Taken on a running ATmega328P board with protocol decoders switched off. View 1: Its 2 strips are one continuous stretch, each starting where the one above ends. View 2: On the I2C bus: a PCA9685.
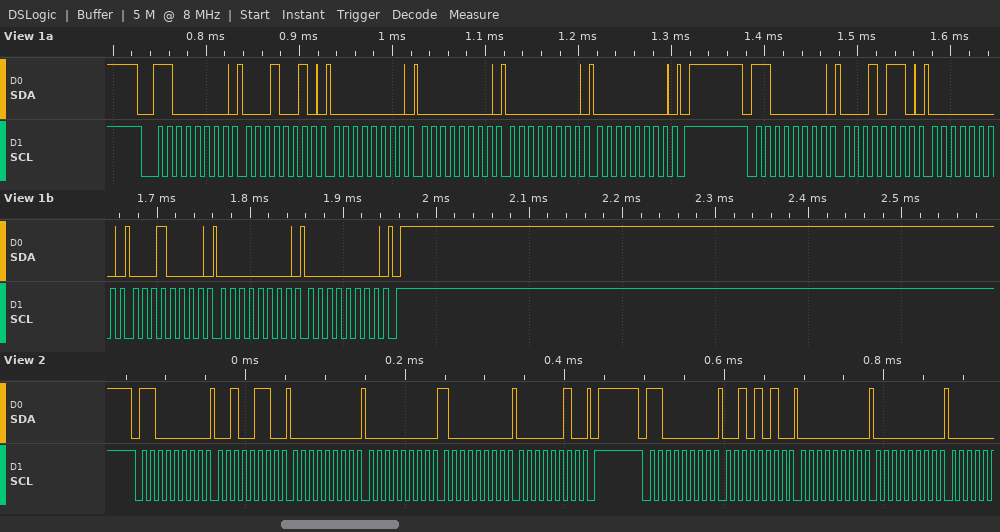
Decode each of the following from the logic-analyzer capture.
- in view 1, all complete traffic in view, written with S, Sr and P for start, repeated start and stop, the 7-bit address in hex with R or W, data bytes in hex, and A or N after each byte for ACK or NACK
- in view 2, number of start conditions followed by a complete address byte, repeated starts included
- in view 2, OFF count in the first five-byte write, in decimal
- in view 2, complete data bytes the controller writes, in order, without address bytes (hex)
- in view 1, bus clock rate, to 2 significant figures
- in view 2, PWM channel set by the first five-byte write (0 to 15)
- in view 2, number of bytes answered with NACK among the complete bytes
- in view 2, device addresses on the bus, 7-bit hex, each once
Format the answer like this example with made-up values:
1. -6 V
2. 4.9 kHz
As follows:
1. S 60W A 12 A 00 A 00 A 00 A 00 A P S 60W A 16 A 00 A 10 A 00 A 00 A P
2. 2
3. 640
4. 26 00 00 80 02 2A 00 00
5. 100 kHz
6. 8
7. 0
8. 0x60
